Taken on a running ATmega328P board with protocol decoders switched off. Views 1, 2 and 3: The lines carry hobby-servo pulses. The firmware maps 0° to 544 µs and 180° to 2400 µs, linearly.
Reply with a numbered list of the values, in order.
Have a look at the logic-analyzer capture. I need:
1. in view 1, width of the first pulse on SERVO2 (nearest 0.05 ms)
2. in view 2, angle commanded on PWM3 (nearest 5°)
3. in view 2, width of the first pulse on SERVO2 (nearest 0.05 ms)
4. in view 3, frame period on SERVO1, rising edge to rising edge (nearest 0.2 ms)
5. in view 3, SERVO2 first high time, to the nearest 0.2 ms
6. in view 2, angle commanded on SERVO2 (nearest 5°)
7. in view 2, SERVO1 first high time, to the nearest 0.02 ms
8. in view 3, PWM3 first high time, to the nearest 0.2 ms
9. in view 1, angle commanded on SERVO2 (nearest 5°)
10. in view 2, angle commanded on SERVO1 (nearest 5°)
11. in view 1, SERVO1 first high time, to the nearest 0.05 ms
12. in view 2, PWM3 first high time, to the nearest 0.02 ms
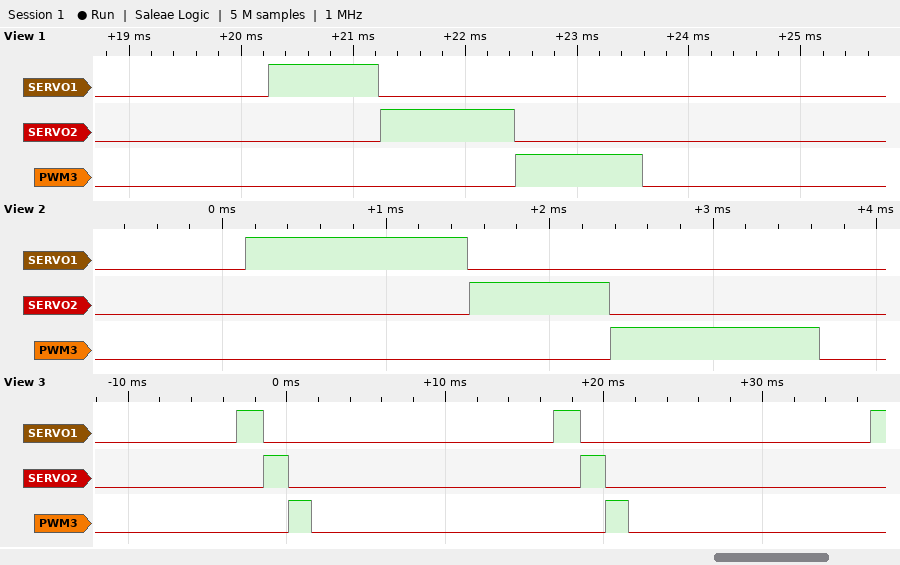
1. 1.20 ms
2. 70°
3. 0.85 ms
4. 20.0 ms
5. 1.6 ms
6. 30°
7. 1.36 ms
8. 1.4 ms
9. 65°
10. 80°
11. 1.00 ms
12. 1.28 ms
